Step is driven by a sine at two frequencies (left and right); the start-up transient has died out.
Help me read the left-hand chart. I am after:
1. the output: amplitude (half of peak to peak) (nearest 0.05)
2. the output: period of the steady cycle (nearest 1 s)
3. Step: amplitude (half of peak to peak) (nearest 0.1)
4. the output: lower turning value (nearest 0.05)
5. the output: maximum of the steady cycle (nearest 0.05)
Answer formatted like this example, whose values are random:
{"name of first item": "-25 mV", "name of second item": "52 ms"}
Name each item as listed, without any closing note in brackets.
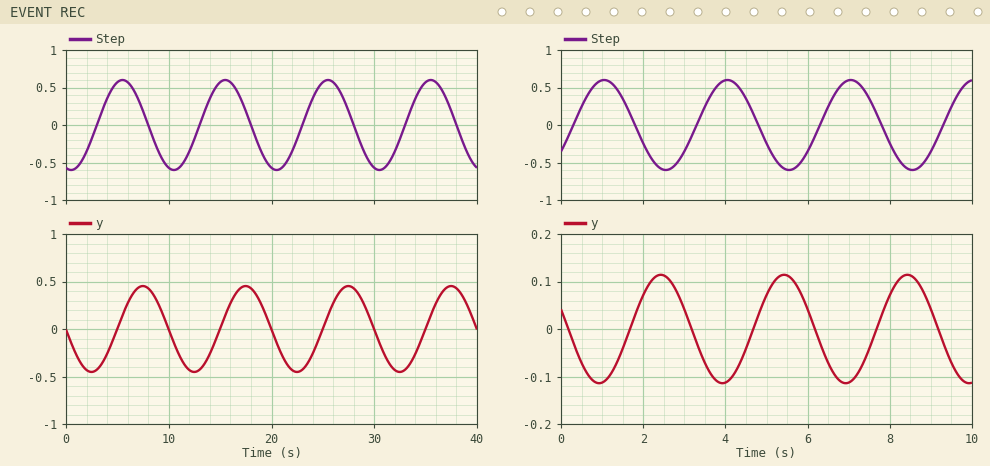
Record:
{"the output: amplitude (half of peak to peak)": "0.45", "the output: period of the steady cycle": "10 s", "Step: amplitude (half of peak to peak)": "0.6", "the output: lower turning value": "-0.45", "the output: maximum of the steady cycle": "0.45"}
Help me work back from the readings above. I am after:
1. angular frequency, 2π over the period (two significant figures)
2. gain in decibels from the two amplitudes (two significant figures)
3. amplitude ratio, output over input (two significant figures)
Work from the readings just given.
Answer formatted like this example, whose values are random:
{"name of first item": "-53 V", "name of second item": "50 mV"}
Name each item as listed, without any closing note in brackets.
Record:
{"angular frequency, 2π over the period": "0.63 rad/s", "gain in decibels from the two amplitudes": "-2.5 dB", "amplitude ratio, output over input": "0.75"}
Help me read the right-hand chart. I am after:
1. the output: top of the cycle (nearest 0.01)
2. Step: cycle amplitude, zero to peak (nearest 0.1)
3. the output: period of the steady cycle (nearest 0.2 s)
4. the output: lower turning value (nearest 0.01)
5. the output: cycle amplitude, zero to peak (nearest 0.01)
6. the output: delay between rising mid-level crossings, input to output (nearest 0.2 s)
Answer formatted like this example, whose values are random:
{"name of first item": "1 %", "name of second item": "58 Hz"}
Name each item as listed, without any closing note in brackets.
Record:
{"the output: top of the cycle": "0.11", "Step: cycle amplitude, zero to peak": "0.6", "the output: period of the steady cycle": "3.0 s", "the output: lower turning value": "-0.11", "the output: cycle amplitude, zero to peak": "0.11", "the output: delay between rising mid-level crossings, input to output": "1.4 s"}
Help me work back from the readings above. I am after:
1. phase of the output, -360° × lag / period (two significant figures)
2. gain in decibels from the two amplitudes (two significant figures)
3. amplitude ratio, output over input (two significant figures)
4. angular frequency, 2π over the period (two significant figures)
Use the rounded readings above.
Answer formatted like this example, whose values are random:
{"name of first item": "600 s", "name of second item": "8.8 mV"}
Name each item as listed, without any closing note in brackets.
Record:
{"phase of the output, -360° × lag / period": "-170°", "gain in decibels from the two amplitudes": "-15 dB", "amplitude ratio, output over input": "0.18", "angular frequency, 2π over the period": "2.1 rad/s"}
